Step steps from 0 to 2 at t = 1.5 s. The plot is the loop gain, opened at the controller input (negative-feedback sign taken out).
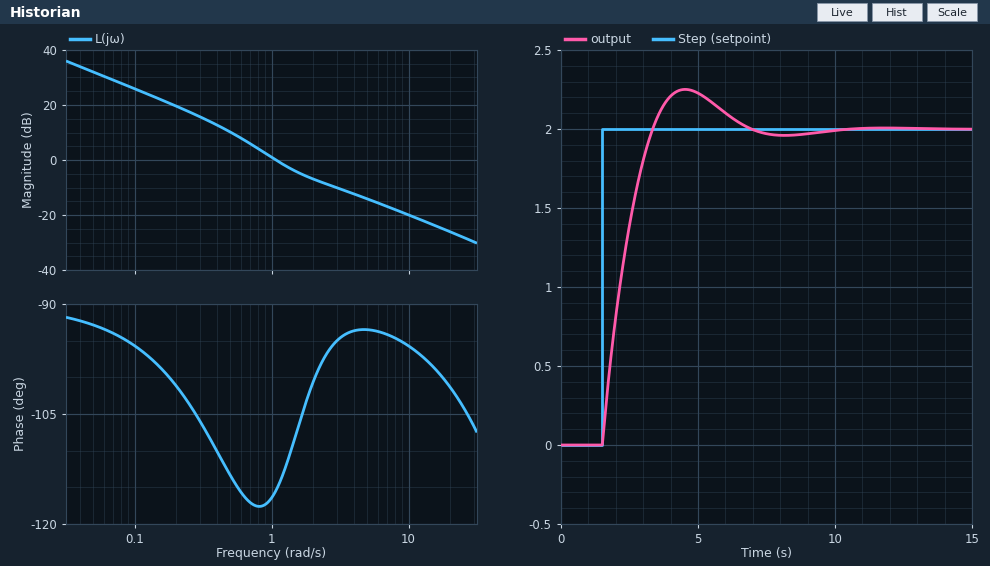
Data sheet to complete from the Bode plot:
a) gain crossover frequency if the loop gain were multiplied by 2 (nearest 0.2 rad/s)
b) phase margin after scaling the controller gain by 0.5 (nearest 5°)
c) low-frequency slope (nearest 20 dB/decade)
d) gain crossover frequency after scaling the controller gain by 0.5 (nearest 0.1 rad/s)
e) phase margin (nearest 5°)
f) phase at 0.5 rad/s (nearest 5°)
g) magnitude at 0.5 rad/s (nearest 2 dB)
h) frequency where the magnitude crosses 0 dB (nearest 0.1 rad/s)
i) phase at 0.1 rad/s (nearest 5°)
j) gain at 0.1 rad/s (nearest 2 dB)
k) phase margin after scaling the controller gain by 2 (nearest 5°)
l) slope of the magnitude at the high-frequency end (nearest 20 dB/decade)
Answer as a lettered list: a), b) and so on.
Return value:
a) 1.8 rad/s
b) 65°
c) -20 dB/decade
d) 0.7 rad/s
e) 65°
f) -115°
g) 10 dB
h) 1.1 rad/s
i) -95°
j) 26 dB
k) 75°
l) -20 dB/decade
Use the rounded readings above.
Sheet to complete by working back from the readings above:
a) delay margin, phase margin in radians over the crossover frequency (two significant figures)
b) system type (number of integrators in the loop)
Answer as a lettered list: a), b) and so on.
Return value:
a) 1.0 s
b) 1
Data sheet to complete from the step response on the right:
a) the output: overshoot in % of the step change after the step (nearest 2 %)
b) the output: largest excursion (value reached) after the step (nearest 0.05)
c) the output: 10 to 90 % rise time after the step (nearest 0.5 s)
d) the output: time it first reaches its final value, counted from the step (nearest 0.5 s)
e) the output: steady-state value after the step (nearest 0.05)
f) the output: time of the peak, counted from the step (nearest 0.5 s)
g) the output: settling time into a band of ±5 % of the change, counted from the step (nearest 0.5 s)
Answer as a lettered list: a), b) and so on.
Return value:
a) 12 %
b) 2.25
c) 1.5 s
d) 2.0 s
e) 2.00
f) 3.0 s
g) 4.5 s
